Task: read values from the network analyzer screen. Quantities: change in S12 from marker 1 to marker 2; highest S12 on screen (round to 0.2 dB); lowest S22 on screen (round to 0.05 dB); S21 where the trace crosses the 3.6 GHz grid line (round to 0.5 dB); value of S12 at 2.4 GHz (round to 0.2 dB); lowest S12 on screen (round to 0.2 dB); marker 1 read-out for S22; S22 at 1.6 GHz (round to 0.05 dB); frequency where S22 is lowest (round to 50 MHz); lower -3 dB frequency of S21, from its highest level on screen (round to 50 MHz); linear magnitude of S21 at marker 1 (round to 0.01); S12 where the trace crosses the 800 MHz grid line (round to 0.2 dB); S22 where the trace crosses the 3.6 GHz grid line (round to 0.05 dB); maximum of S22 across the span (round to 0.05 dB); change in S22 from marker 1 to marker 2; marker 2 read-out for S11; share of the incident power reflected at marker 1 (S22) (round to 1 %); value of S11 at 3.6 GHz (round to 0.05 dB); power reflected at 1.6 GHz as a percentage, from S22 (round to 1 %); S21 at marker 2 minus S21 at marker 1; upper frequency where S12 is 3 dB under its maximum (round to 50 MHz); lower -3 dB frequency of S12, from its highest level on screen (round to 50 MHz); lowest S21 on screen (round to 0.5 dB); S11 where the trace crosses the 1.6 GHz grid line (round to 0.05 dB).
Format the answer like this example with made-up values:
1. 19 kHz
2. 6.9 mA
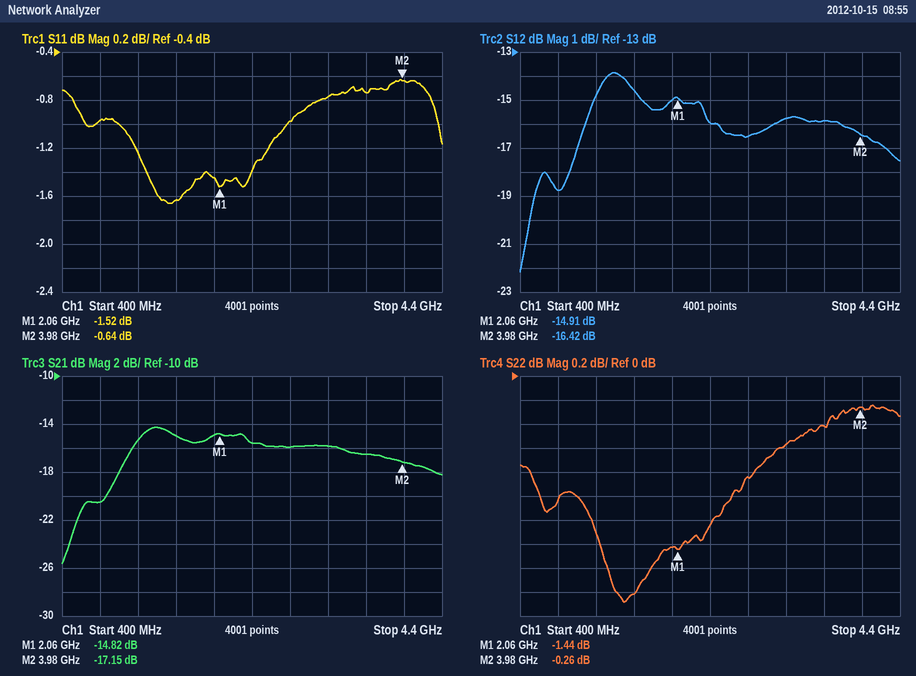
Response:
1. -1.51 dB
2. -13.8 dB
3. -1.90 dB
4. -16.5 dB
5. -16.0 dB
6. -22.2 dB
7. -1.44 dB
8. -1.80 dB
9. 1.50 GHz
10. 1.05 GHz
11. 0.18
12. -18.8 dB
13. -0.40 dB
14. -0.25 dB
15. 1.18 dB
16. -0.64 dB
17. 72 %
18. -0.75 dB
19. 66 %
20. -2.33 dB
21. 4.20 GHz
22. 1.00 GHz
23. -25.5 dB
24. -1.65 dB
